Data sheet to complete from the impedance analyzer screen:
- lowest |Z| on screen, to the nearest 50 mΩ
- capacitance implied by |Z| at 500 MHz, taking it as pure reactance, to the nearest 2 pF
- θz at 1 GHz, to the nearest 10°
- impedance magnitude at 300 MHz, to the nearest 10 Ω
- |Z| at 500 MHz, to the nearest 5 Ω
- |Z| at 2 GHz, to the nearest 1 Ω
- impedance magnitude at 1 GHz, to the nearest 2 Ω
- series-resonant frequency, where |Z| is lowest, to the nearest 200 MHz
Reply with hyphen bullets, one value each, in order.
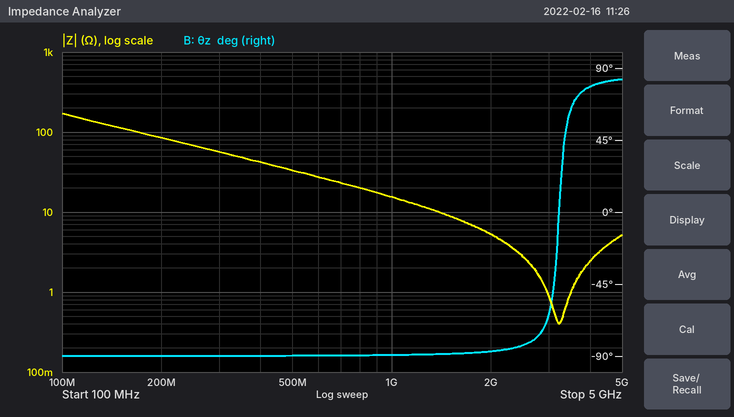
- 400 mΩ
- 10 pF
- -90°
- 60 Ω
- 35 Ω
- 5 Ω
- 16 Ω
- 3.2 GHz
